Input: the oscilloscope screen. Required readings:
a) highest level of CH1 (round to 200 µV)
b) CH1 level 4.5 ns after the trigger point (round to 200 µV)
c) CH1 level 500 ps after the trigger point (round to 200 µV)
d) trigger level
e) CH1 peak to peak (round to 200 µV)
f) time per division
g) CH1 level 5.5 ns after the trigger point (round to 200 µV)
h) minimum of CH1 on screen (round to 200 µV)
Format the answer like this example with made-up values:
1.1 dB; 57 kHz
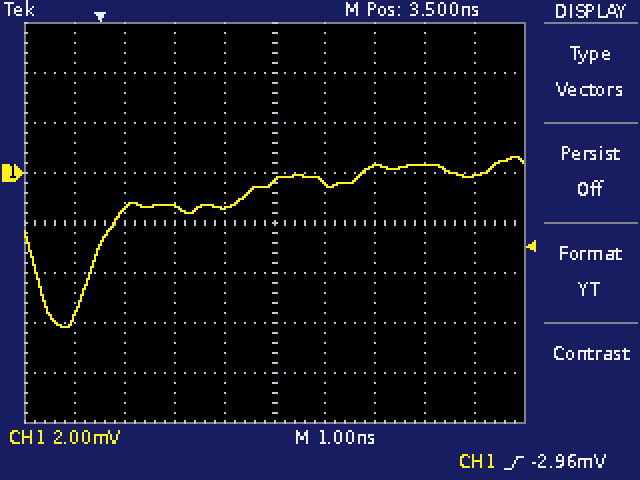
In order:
600 µV; -400 µV; -1.4 mV; -2.96 mV; 6.8 mV; 1 ns; 200 µV; -6.2 mV
